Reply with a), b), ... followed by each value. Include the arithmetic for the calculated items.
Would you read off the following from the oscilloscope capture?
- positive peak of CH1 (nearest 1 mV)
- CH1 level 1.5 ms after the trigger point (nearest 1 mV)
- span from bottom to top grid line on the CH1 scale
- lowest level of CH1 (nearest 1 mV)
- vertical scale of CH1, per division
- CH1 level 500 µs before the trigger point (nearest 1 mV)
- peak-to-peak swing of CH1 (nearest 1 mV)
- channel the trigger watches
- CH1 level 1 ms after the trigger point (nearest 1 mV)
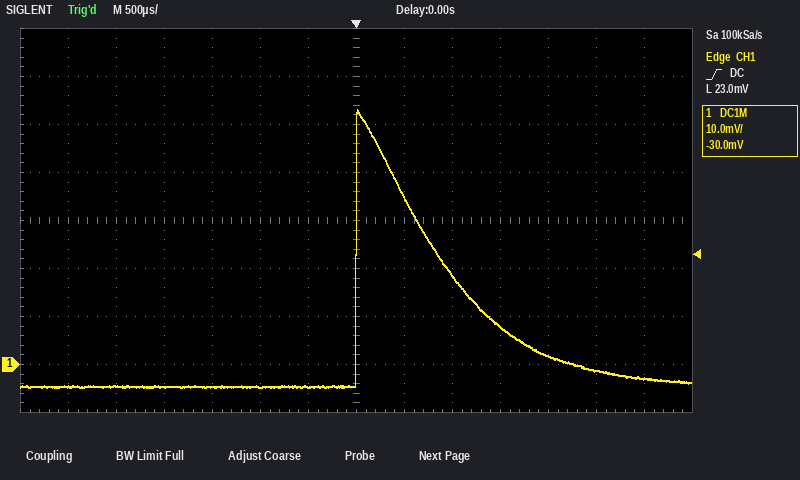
a) 53 mV
b) 8 mV
c) 80 mV
d) -5 mV
e) 10 mV
f) -5 mV
g) 53 mV − (-5 mV) = 58 mV
h) CH1
i) 19 mV
